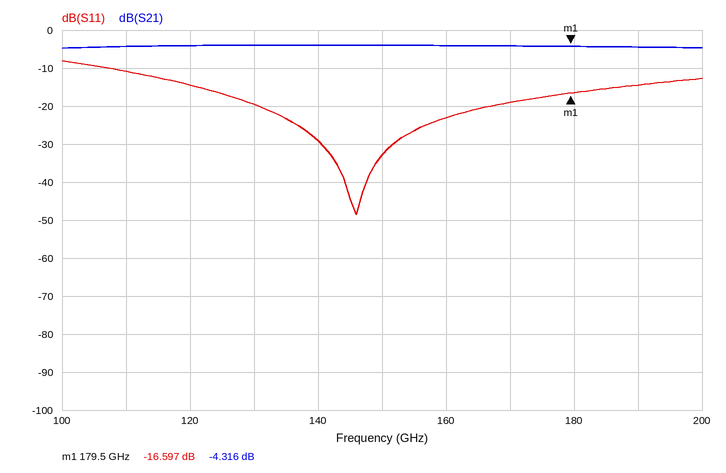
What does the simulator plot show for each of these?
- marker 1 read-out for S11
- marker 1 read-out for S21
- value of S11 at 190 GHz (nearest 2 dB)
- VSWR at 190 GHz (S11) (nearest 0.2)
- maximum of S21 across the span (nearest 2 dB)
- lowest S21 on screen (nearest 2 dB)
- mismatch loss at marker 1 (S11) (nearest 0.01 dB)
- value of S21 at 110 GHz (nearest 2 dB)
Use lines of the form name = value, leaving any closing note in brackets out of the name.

marker 1 read-out for S11 = -16.597 dB
marker 1 read-out for S21 = -4.316 dB
value of S11 at 190 GHz = -14 dB
VSWR at 190 GHz (S11) = 1.4
maximum of S21 across the span = -4 dB
lowest S21 on screen = -4 dB
mismatch loss at marker 1 (S11) = 0.10 dB
value of S21 at 110 GHz = -4 dB
